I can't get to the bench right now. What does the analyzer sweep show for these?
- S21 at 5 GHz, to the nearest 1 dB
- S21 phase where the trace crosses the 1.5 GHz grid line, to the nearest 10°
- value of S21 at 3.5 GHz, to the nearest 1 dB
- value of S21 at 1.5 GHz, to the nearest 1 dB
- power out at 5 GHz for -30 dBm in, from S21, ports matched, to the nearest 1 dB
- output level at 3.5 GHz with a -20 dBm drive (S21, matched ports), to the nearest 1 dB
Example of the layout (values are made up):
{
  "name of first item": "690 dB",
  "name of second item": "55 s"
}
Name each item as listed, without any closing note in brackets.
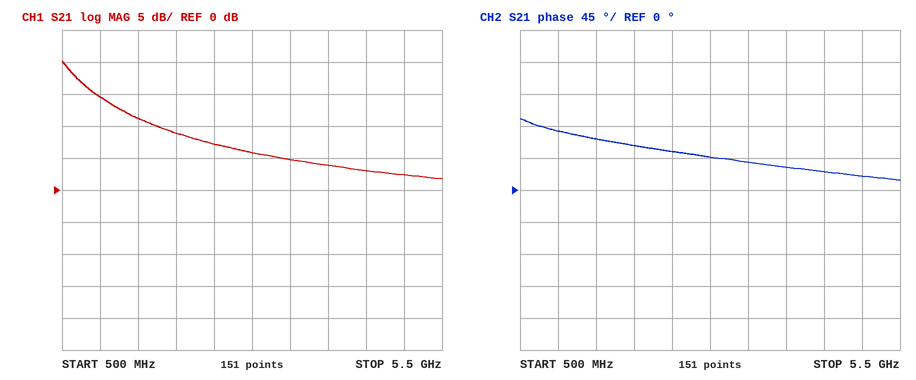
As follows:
{
  "S21 at 5 GHz, to the nearest 1 dB": "2 dB",
  "S21 phase where the trace crosses the 1.5 GHz grid line, to the nearest 10°": "70°",
  "value of S21 at 3.5 GHz, to the nearest 1 dB": "5 dB",
  "value of S21 at 1.5 GHz, to the nearest 1 dB": "11 dB",
  "power out at 5 GHz for -30 dBm in, from S21, ports matched, to the nearest 1 dB": "-28 dBm",
  "output level at 3.5 GHz with a -20 dBm drive (S21, matched ports), to the nearest 1 dB": "-15 dBm"
}
